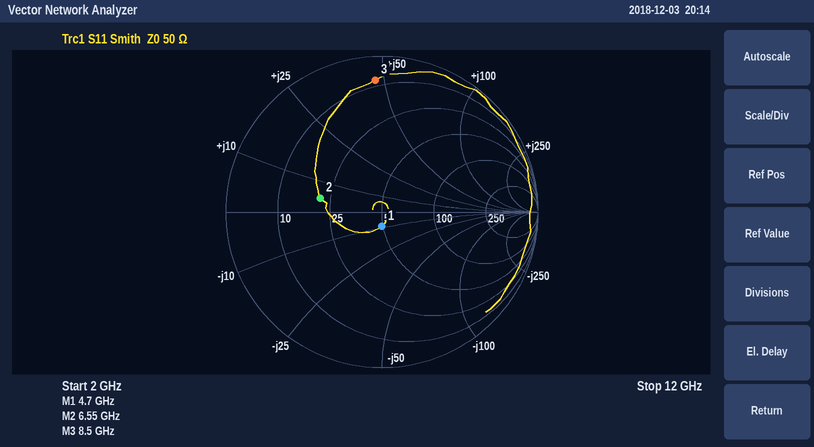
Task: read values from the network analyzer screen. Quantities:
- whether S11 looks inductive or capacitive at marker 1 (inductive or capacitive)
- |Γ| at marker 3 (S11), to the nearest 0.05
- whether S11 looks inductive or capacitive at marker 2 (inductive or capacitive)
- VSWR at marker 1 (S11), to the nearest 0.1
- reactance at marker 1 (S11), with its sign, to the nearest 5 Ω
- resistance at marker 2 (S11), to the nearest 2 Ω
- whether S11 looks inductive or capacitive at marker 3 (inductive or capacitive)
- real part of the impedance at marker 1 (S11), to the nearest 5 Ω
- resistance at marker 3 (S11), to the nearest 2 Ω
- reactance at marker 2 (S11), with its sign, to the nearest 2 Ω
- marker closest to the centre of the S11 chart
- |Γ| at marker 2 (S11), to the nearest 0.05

capacitive
0.85
inductive
1.2
-10 Ω
22 Ω
inductive
50 Ω
8 Ω
+4 Ω
marker 1
0.40
